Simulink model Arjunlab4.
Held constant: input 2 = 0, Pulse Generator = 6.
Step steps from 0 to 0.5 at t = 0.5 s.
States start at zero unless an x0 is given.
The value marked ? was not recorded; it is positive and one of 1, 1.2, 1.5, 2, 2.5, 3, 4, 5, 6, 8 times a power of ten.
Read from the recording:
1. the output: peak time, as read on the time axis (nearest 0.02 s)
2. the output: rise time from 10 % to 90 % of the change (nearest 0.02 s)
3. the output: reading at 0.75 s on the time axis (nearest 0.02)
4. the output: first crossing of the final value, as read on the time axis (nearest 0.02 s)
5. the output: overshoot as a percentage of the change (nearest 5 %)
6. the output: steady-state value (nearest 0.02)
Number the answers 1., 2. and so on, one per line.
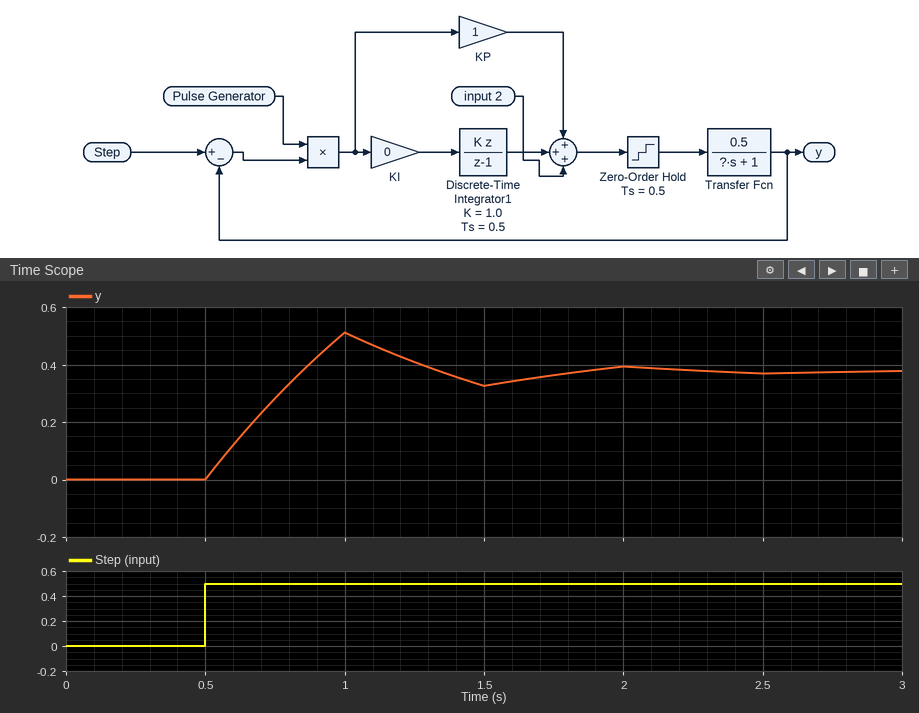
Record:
1. 1.00 s
2. 0.28 s
3. 0.28
4. 0.84 s
5. 35 %
6. 0.38
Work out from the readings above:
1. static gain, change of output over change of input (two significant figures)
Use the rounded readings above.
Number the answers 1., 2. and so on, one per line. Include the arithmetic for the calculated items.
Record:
1. (0.38 - 0) / (0.5 - 0) = 0.76
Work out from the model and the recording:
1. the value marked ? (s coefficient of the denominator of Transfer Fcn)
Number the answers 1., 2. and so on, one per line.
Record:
1. 1.2
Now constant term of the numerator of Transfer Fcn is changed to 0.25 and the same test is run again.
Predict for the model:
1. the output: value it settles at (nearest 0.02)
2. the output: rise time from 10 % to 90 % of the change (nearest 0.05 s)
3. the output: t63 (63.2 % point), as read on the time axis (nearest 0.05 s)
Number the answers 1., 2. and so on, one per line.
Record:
1. 0.30
2. 0.60 s
3. 0.85 s
